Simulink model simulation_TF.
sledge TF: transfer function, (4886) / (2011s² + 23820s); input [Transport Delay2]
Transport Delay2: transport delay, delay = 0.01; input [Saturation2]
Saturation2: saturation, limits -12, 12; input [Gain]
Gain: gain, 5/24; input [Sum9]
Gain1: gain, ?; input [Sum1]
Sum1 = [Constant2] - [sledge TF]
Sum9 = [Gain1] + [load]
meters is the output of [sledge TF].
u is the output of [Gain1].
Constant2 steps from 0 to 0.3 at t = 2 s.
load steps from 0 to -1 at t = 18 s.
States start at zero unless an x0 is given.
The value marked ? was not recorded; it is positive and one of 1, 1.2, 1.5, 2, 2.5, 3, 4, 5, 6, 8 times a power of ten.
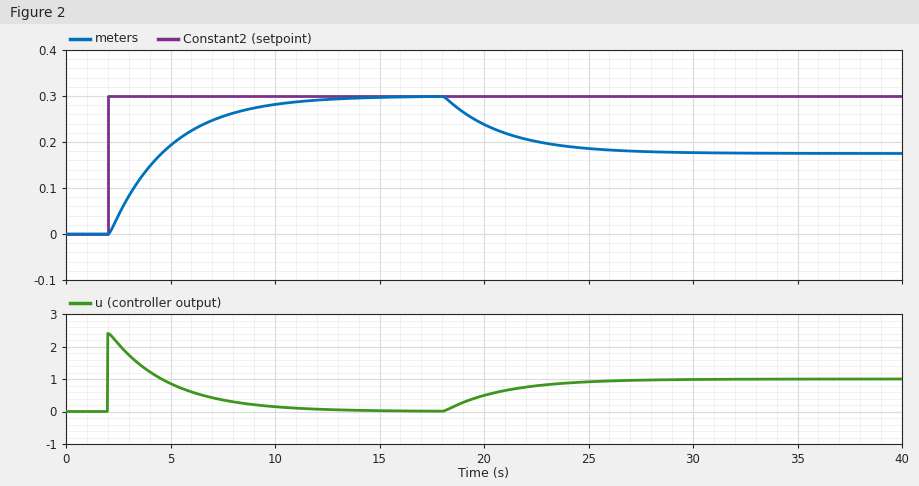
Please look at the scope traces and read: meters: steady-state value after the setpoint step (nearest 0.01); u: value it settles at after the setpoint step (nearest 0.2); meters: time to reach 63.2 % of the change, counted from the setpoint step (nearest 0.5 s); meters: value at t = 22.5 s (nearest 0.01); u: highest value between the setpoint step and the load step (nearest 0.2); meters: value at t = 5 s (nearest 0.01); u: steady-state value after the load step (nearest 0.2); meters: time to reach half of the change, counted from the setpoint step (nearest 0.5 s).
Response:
0.30
0.0
3.0 s
0.20
2.4
0.19
1.0
2.0 s
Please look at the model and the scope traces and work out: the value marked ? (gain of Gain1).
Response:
8
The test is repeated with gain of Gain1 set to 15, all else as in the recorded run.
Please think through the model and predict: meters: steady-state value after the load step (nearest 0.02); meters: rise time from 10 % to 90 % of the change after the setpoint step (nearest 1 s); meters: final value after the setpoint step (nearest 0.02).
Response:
0.24
3 s
0.30
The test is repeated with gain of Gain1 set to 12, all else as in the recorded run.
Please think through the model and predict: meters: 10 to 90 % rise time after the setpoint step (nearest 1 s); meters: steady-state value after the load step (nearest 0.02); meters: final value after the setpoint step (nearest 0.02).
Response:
4 s
0.22
0.30
